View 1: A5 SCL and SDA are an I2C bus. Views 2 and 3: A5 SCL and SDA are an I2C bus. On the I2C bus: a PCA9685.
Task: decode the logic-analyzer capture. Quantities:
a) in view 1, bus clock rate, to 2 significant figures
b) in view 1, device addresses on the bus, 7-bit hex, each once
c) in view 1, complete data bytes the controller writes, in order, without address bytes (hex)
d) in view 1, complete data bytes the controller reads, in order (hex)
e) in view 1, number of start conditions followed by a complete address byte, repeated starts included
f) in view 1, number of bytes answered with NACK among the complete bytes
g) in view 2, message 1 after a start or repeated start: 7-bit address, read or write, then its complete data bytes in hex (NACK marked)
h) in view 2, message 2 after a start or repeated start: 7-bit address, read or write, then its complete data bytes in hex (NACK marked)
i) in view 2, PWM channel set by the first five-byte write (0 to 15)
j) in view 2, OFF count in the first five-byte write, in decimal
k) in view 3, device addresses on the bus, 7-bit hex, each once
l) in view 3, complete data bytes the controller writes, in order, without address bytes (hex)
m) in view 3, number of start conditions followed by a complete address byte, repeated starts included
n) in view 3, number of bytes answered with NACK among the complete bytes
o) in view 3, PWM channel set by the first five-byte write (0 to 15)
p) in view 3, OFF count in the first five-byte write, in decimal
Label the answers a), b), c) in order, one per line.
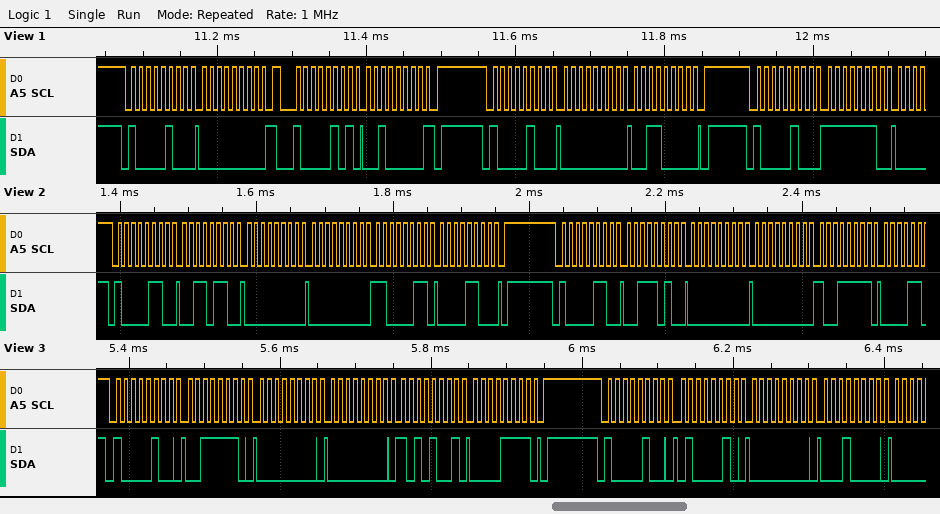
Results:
a) 100 kHz
b) 0x42
c) 00 00 30 FE
d) 20
e) 4
f) 1
g) 0x43 write: 36 00 00 C3 0C
h) 0x43 write: 3A 00 00 9F
i) 12
j) 3267
k) 0x42
l) 3E 00 00 A9 0F 42 00 10
m) 2
n) 0
o) 14
p) 4009
